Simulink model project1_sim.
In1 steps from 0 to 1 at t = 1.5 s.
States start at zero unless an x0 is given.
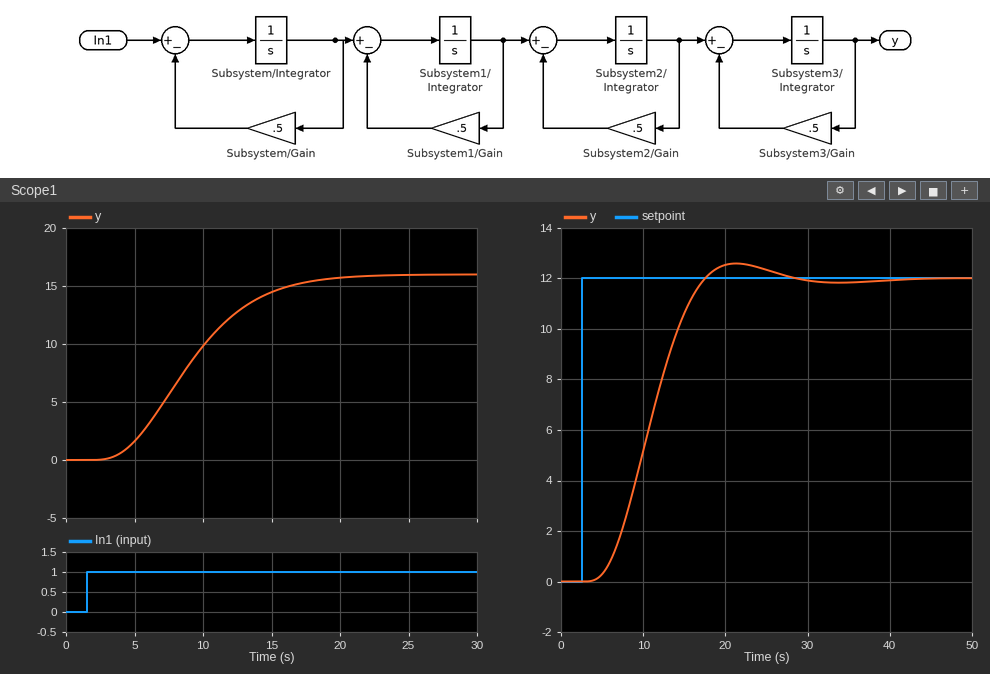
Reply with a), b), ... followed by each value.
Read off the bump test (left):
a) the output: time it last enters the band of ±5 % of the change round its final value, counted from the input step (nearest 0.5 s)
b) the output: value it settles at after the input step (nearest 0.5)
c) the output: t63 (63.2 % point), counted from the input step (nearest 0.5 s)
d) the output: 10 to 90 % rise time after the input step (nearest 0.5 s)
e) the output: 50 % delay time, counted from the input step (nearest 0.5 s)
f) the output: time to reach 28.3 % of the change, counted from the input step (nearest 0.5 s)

a) 15.5 s
b) 16.0
c) 8.5 s
d) 10.0 s
e) 7.5 s
f) 5.5 s
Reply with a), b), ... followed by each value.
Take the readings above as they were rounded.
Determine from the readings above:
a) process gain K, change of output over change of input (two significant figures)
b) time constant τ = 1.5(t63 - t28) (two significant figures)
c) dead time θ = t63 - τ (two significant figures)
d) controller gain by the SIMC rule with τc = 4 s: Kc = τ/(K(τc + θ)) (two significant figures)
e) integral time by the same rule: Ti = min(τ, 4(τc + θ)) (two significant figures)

a) 16
b) 4.5 s
c) 4.0 s
d) 0.035
e) 4.5 s
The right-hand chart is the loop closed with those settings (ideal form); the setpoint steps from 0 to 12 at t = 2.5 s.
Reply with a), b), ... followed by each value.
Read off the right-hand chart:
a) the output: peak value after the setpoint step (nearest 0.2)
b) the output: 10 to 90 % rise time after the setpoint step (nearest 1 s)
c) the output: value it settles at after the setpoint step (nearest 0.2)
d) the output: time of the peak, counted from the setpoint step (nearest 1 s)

a) 12.6
b) 9 s
c) 12.0
d) 19 s
